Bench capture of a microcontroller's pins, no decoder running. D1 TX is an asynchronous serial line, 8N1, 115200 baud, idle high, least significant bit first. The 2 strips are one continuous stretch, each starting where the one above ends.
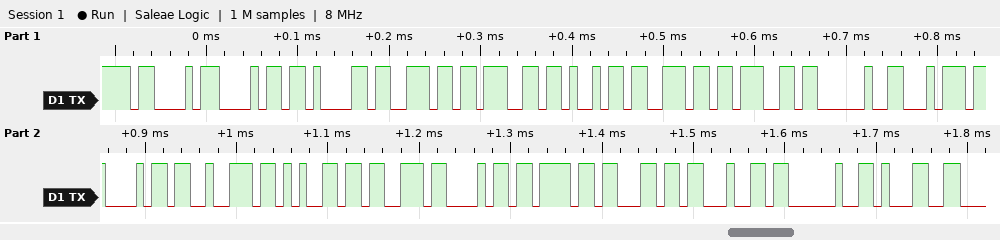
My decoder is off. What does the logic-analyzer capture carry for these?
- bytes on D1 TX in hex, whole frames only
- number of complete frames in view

43 68 61 6E 67 69 6E 67 20 74 68 72 65 73 68 6F 6C 64 20 31
20
